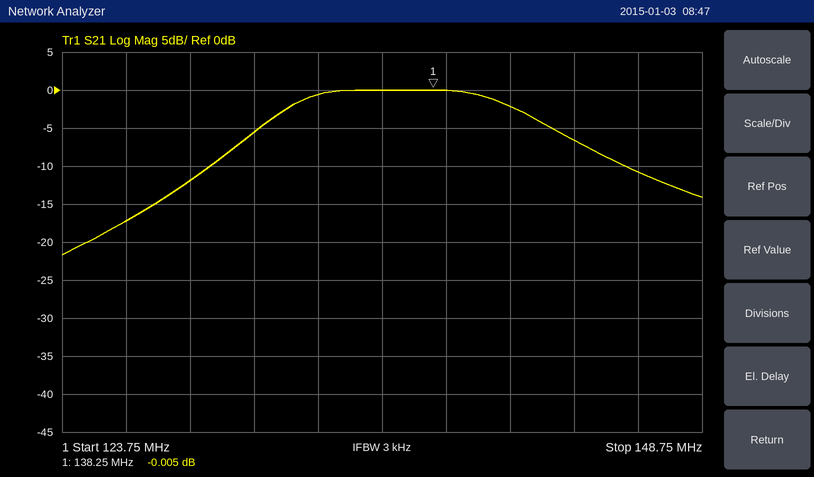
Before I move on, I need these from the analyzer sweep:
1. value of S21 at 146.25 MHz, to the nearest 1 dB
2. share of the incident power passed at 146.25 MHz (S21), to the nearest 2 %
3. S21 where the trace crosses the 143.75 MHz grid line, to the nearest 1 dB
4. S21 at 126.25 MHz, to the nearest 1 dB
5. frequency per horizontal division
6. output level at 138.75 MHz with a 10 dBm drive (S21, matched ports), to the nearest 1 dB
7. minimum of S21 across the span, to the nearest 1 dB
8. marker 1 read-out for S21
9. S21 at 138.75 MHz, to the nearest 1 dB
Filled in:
-11 dB
8 %
-7 dB
-17 dB
2.5 MHz
10 dBm
-22 dB
-0.005 dB
0 dB
